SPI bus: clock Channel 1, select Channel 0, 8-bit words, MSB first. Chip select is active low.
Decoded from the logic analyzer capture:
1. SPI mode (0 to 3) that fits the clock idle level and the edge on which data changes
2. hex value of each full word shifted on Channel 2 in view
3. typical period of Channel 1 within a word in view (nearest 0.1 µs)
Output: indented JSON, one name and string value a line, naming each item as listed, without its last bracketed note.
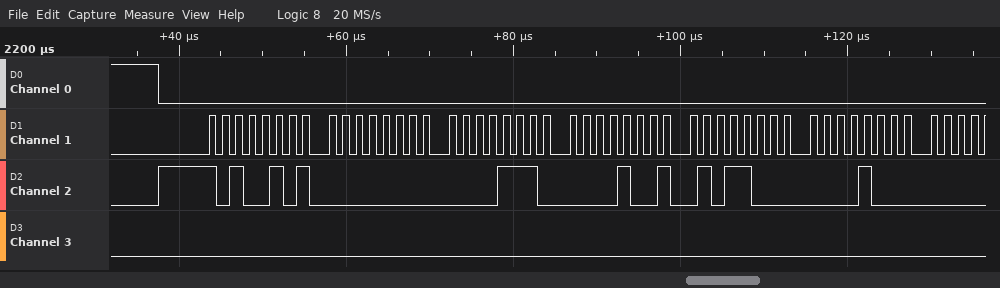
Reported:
{
  "SPI mode (0 to 3) that fits the clock idle level and the edge on which data changes": "0",
  "hex value of each full word shifted on Channel 2 in view": "A5, 00, 0E, 09, 58, 08",
  "typical period of Channel 1 within a word in view": "1.6 µs"
}
